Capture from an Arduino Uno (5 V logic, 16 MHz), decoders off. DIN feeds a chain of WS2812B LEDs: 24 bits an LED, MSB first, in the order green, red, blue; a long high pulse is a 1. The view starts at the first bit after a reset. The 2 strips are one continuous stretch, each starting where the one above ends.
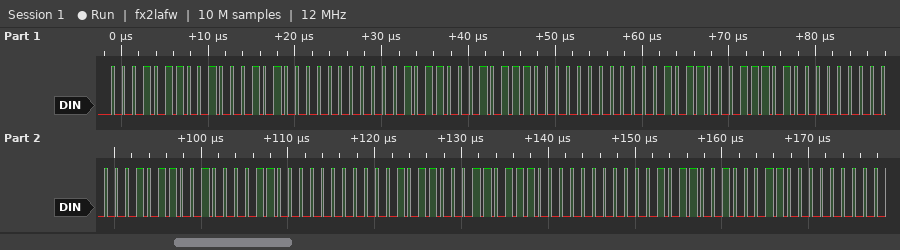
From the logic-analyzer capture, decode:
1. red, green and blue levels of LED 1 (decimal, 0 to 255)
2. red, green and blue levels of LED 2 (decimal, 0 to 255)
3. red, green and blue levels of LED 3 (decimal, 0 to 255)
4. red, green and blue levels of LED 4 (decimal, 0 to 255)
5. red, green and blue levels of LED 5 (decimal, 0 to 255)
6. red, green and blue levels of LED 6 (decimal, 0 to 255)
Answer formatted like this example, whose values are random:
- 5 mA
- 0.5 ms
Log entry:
- 69, 22, 0
- 46, 22, 0
- 58, 22, 0
- 67, 22, 0
- 55, 22, 0
- 70, 22, 0
